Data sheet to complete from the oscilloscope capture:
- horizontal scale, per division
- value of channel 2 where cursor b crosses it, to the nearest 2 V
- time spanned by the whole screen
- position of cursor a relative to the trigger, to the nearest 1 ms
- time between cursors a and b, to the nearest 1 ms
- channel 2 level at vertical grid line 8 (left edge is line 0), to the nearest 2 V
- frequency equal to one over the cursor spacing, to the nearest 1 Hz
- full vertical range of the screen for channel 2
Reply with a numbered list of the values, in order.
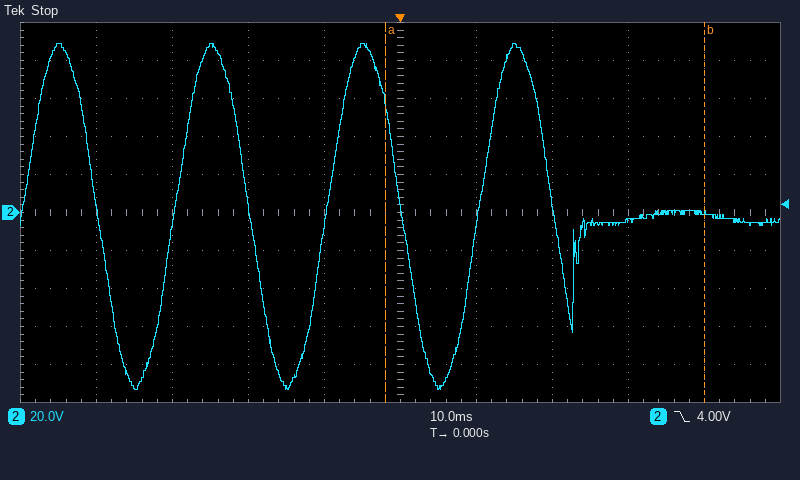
1. 10 ms
2. 0 V
3. 100 ms
4. -2 ms
5. 42 ms
6. -4 V
7. 24 Hz
8. 200 V
